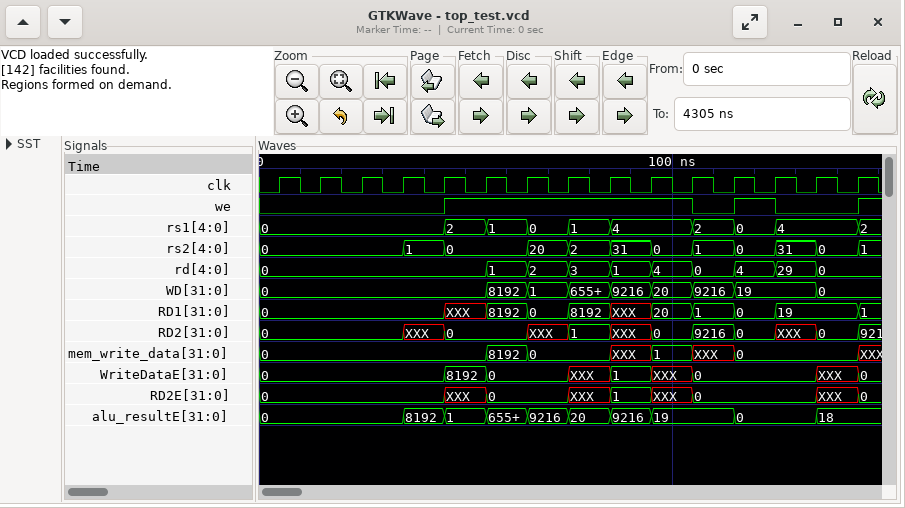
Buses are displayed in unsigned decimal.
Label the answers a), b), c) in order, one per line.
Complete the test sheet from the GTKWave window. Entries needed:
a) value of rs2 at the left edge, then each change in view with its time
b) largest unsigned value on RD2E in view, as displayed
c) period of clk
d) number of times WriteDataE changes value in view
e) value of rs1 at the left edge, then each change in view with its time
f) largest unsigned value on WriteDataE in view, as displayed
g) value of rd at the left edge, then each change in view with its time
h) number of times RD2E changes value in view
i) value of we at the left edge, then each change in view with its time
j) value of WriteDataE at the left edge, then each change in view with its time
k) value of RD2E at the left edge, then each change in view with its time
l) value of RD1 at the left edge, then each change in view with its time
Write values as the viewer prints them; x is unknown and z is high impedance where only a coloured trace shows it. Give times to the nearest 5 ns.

a) 0, 1 at 35 ns, 0 at 45 ns, 20 at 65 ns, 2 at 75 ns, 31 at 85 ns, 0 at 95 ns, 1 at 105 ns, 0 at 115 ns, 31 at 125 ns, 0 at 135 ns, 1 at 145 ns
b) 1
c) 10 ns
d) 8
e) 0, 2 at 45 ns, 1 at 55 ns, 0 at 65 ns, 1 at 75 ns, 4 at 85 ns, 2 at 105 ns, 0 at 115 ns, 4 at 125 ns, 2 at 145 ns
f) 8192
g) 0, 1 at 55 ns, 2 at 65 ns, 3 at 75 ns, 1 at 85 ns, 4 at 95 ns, 0 at 105 ns, 4 at 115 ns, 29 at 125 ns, 0 at 135 ns
h) 8
i) 0, 1 at 45 ns, 0 at 105 ns, 1 at 115 ns, 0 at 125 ns, 1 at 145 ns
j) 0, 8192 at 45 ns, 0 at 55 ns, XXX at 75 ns, 1 at 85 ns, XXX at 95 ns, 0 at 105 ns, XXX at 135 ns, 0 at 145 ns
k) 0, XXX at 45 ns, 0 at 55 ns, XXX at 75 ns, 1 at 85 ns, XXX at 95 ns, 0 at 105 ns, XXX at 135 ns, 0 at 145 ns
l) 0, XXX at 45 ns, 8192 at 55 ns, 0 at 65 ns, 8192 at 75 ns, XXX at 85 ns, 20 at 95 ns, 1 at 105 ns, 0 at 115 ns, 19 at 125 ns, 1 at 145 ns
